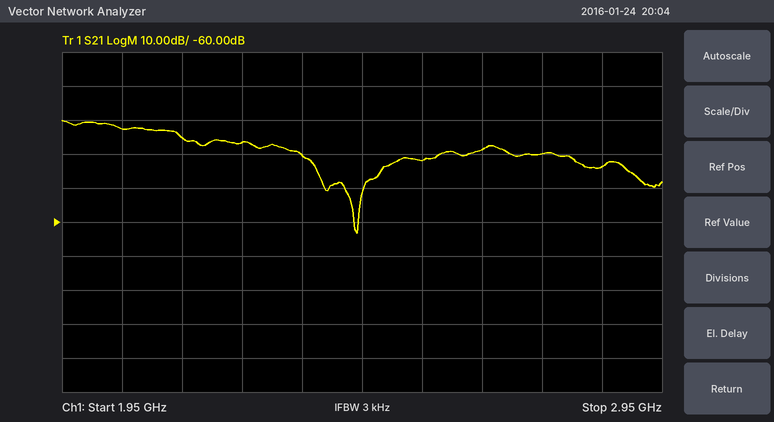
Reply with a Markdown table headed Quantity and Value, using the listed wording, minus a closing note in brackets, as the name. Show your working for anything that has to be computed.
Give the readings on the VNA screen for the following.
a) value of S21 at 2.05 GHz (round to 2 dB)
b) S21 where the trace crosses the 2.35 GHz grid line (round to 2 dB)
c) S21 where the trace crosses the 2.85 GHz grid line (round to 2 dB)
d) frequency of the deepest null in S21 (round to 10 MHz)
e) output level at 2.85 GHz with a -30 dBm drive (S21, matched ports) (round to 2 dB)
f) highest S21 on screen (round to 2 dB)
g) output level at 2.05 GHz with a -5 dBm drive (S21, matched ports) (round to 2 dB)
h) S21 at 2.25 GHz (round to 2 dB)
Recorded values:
| Quantity | Value |
|---|---|
| value of S21 at 2.05 GHz | -32 dB |
| S21 where the trace crosses the 2.35 GHz grid line | -40 dB |
| S21 where the trace crosses the 2.85 GHz grid line | -44 dB |
| frequency of the deepest null in S21 | 2.44 GHz |
| output level at 2.85 GHz with a -30 dBm drive (S21, matched ports) | -30 dBm + (-44 dB) = -74 dBm |
| highest S21 on screen | -30 dB |
| output level at 2.05 GHz with a -5 dBm drive (S21, matched ports) | -5 dBm + (-32 dB) = -38 dBm |
| S21 at 2.25 GHz | -36 dB |
